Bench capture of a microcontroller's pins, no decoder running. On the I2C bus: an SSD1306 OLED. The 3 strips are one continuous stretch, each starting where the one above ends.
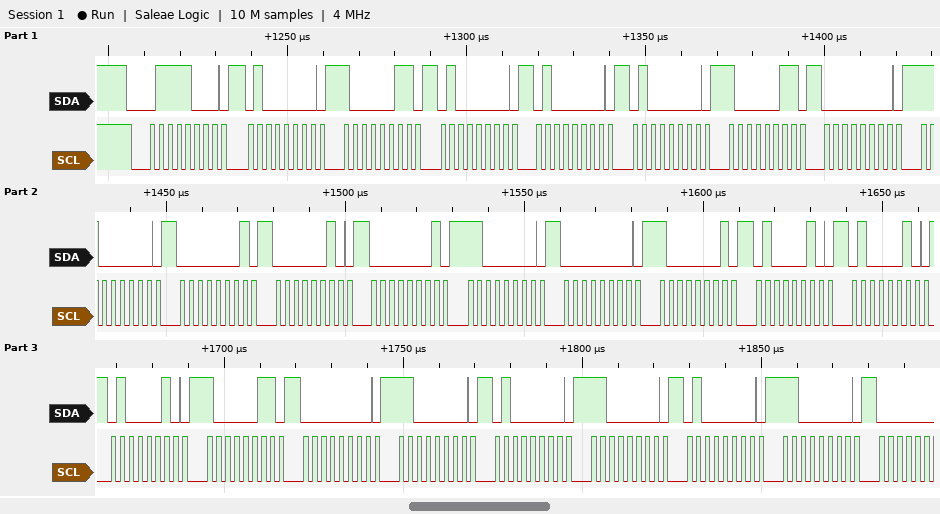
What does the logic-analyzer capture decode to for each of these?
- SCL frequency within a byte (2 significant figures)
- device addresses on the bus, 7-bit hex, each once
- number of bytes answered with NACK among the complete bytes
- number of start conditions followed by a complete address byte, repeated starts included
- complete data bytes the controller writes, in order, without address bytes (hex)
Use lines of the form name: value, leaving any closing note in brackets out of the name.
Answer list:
SCL frequency within a byte: 400 kHz
device addresses on the bus, 7-bit hex, each once: 0x3C
number of bytes answered with NACK among the complete bytes: 0
number of start conditions followed by a complete address byte, repeated starts included: 1
complete data bytes the controller writes, in order, without address bytes: 40 83 40 40 40 83 00 C0 01 02 01 C0 00 81 42 42 42 83 00 C0 40 C0 40 C0
